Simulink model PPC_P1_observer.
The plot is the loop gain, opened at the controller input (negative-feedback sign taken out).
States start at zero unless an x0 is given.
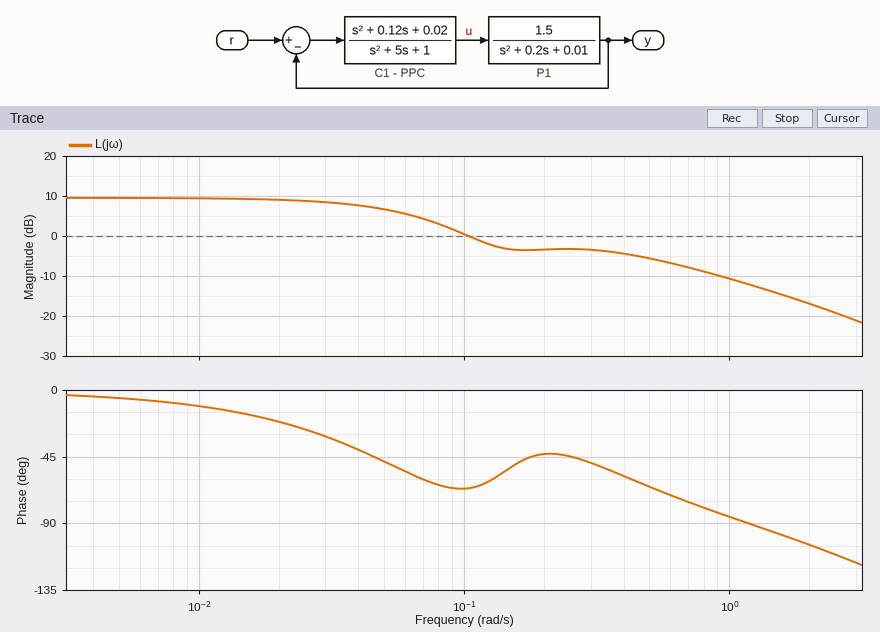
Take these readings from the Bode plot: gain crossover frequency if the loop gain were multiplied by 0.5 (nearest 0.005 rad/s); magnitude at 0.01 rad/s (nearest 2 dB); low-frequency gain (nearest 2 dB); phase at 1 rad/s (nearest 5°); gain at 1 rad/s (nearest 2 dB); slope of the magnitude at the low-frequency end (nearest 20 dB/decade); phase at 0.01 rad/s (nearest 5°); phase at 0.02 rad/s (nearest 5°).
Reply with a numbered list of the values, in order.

1. 0.055 rad/s
2. 10 dB
3. 10 dB
4. -85°
5. -10 dB
6. 0 dB/decade
7. -10°
8. -20°
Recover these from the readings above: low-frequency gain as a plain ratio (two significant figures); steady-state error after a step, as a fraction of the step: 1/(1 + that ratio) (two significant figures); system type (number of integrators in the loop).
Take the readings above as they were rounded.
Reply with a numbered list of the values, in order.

1. 3.2
2. 0.24
3. 0
